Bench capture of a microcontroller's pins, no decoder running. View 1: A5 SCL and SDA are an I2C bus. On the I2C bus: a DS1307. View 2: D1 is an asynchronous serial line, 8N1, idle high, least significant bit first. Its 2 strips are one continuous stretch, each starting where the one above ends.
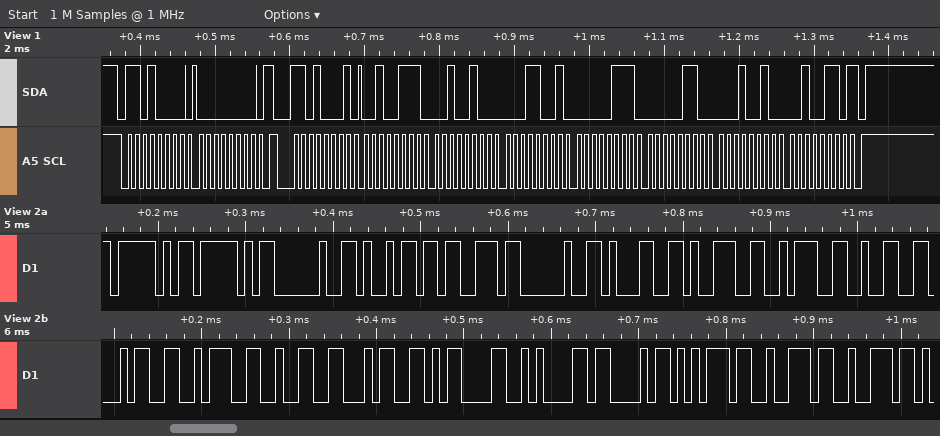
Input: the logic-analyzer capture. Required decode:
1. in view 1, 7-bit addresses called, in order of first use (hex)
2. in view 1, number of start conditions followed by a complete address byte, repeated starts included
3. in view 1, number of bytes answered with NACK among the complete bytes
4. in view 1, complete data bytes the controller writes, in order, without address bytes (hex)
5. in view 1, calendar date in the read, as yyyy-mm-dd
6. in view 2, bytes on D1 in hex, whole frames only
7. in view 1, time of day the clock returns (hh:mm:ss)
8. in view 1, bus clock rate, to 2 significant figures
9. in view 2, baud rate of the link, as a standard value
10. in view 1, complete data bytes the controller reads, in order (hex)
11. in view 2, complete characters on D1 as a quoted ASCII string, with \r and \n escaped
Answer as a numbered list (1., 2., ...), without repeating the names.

1. 0x68
2. 2
3. 1
4. 00
5. 2026-12-06
6. 5F 5F 20 69 73 20 31 39 3A 32 34 3A 32 34 0D 0A 43 75 72 72
7. 19:24:27
8. 100 kHz
9. 115200 baud
10. 27 24 19 07 06 12 26
11. "__ is 19:24:24\r\nCurr"
